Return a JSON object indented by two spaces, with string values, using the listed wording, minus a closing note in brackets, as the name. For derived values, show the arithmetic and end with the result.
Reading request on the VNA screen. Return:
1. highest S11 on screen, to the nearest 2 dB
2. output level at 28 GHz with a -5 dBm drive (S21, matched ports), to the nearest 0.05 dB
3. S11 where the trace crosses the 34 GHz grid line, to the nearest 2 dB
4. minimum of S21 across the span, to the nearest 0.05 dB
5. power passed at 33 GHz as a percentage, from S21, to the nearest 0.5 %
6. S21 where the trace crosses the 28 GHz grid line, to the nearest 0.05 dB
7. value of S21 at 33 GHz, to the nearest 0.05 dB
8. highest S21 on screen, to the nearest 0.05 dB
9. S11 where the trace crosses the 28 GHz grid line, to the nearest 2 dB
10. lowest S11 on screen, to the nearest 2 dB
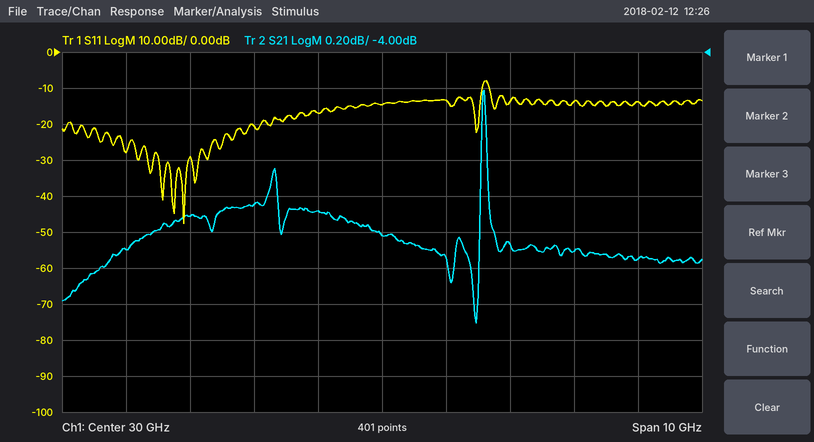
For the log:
{
  "highest S11 on screen, to the nearest 2 dB": "-8 dB",
  "output level at 28 GHz with a -5 dBm drive (S21, matched ports), to the nearest 0.05 dB": "-5 dBm + (-4.85 dB) = -9.85 dBm",
  "S11 where the trace crosses the 34 GHz grid line, to the nearest 2 dB": "-14 dB",
  "minimum of S21 across the span, to the nearest 0.05 dB": "-5.50 dB",
  "power passed at 33 GHz as a percentage, from S21, to the nearest 0.5 %": "10^(-5.1/10) ≈ 30.9 %, so 31.0 % to the nearest 0.5 %",
  "S21 where the trace crosses the 28 GHz grid line, to the nearest 0.05 dB": "-4.85 dB",
  "value of S21 at 33 GHz, to the nearest 0.05 dB": "-5.10 dB",
  "highest S21 on screen, to the nearest 0.05 dB": "-4.20 dB",
  "S11 where the trace crosses the 28 GHz grid line, to the nearest 2 dB": "-20 dB",
  "lowest S11 on screen, to the nearest 2 dB": "-48 dB"
}
